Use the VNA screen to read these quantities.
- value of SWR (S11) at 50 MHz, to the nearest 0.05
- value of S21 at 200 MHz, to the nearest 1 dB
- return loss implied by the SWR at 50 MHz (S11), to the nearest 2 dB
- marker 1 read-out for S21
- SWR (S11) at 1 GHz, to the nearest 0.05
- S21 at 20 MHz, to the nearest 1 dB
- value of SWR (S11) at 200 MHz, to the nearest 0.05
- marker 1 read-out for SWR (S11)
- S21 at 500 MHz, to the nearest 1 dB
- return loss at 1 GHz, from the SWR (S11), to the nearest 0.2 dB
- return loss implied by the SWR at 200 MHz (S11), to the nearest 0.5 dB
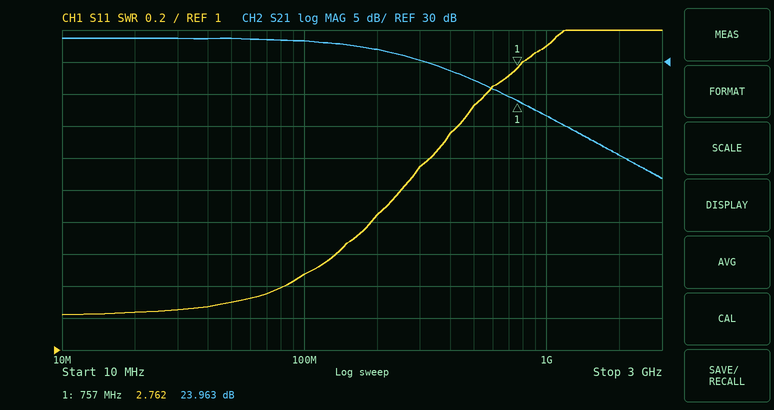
1.30
32 dB
18 dB
23.963 dB
2.90
34 dB
1.85
2.762
27 dB
6.2 dB
10.5 dB
